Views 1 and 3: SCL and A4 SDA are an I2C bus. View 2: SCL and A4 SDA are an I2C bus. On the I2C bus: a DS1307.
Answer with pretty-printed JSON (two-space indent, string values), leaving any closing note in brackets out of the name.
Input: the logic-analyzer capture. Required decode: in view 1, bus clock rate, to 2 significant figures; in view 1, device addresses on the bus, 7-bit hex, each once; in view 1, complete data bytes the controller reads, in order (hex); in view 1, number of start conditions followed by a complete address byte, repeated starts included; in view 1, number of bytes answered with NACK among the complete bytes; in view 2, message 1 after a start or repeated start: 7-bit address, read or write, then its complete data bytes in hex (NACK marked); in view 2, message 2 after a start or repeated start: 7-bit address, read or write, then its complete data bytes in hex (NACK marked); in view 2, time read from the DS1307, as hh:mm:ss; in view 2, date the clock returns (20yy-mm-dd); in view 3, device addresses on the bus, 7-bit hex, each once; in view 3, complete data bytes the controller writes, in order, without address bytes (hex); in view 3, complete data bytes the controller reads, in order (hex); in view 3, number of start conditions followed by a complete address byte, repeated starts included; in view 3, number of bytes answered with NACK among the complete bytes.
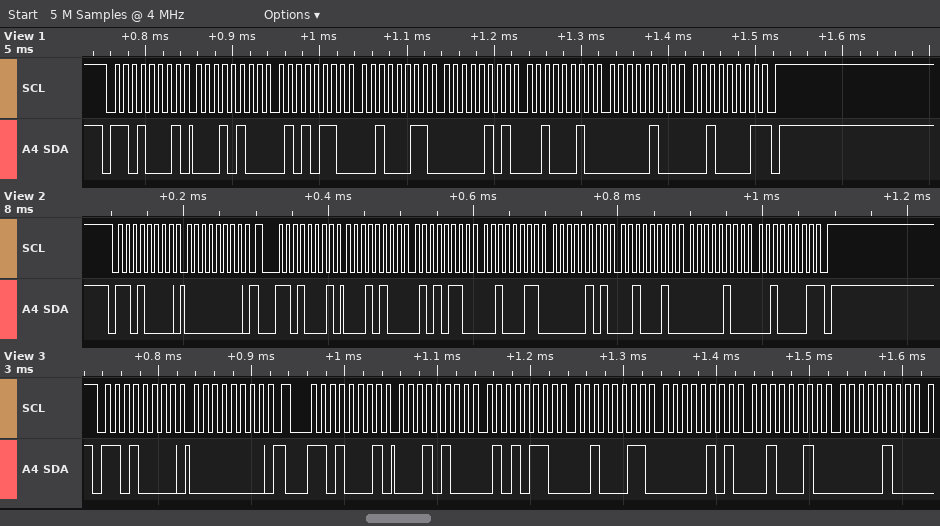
{
  "in view 1, bus clock rate, to 2 significant figures": "100 kHz",
  "in view 1, device addresses on the bus, 7-bit hex, each once": "0x68",
  "in view 1, complete data bytes the controller reads, in order": "14 56 23 05 22 04 21",
  "in view 1, number of start conditions followed by a complete address byte, repeated starts included": "1",
  "in view 1, number of bytes answered with NACK among the complete bytes": "1",
  "in view 2, message 1 after a start or repeated start: 7-bit address, read or write, then its complete data bytes in hex": "0x68 write: 00",
  "in view 2, message 2 after a start or repeated start: 7-bit address, read or write, then its complete data bytes in hex": "0x68 read: 14 56 23 05 22 04 21 NACK",
  "in view 2, time read from the DS1307, as hh:mm:ss": "23:56:14",
  "in view 2, date the clock returns": "2021-04-22",
  "in view 3, device addresses on the bus, 7-bit hex, each once": "0x68",
  "in view 3, complete data bytes the controller writes, in order, without address bytes": "00",
  "in view 3, complete data bytes the controller reads, in order": "14 56 23 05 22 04",
  "in view 3, number of start conditions followed by a complete address byte, repeated starts included": "2",
  "in view 3, number of bytes answered with NACK among the complete bytes": "0"
}
